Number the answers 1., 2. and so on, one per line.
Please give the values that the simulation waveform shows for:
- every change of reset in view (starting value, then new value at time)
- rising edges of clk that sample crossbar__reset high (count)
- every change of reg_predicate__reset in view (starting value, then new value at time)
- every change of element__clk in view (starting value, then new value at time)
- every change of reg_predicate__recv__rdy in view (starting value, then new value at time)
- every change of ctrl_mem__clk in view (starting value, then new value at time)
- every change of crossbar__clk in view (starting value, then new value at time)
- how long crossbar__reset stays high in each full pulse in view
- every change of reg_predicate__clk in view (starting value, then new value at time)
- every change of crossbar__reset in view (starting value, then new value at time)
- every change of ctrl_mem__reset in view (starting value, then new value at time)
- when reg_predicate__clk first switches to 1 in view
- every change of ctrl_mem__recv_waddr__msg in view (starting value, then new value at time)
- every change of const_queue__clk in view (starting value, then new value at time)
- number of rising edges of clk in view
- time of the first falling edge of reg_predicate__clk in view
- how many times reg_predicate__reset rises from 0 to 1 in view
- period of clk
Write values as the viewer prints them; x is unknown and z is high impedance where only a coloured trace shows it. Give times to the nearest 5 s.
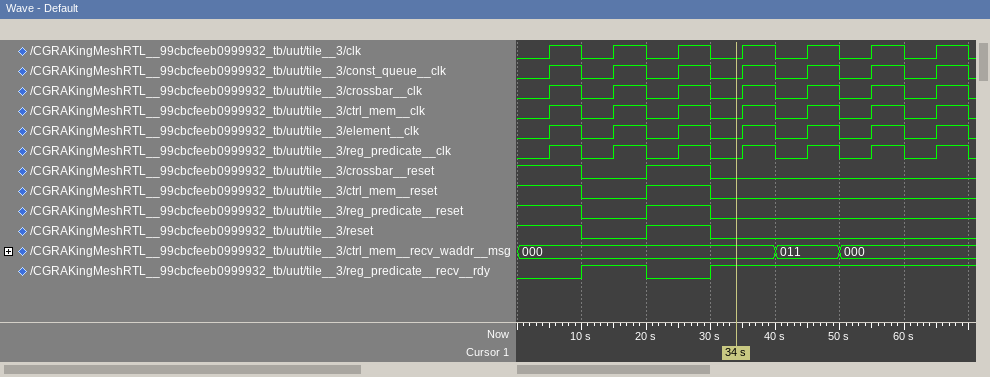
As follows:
1. 1, 0 at 10 s, 1 at 20 s, 0 at 30 s
2. 2
3. 1, 0 at 10 s, 1 at 20 s, 0 at 30 s
4. 0, 1 at 5 s, 0 at 10 s, 1 at 15 s, 0 at 20 s, 1 at 25 s, 0 at 30 s, 1 at 35 s, 0 at 40 s, 1 at 45 s, 0 at 50 s, 1 at 55 s, 0 at 60 s, 1 at 65 s, 0 at 70 s
5. 0, 1 at 10 s, 0 at 20 s, 1 at 30 s
6. 0, 1 at 5 s, 0 at 10 s, 1 at 15 s, 0 at 20 s, 1 at 25 s, 0 at 30 s, 1 at 35 s, 0 at 40 s, 1 at 45 s, 0 at 50 s, 1 at 55 s, 0 at 60 s, 1 at 65 s, 0 at 70 s
7. 0, 1 at 5 s, 0 at 10 s, 1 at 15 s, 0 at 20 s, 1 at 25 s, 0 at 30 s, 1 at 35 s, 0 at 40 s, 1 at 45 s, 0 at 50 s, 1 at 55 s, 0 at 60 s, 1 at 65 s, 0 at 70 s
8. 10 s
9. 0, 1 at 5 s, 0 at 10 s, 1 at 15 s, 0 at 20 s, 1 at 25 s, 0 at 30 s, 1 at 35 s, 0 at 40 s, 1 at 45 s, 0 at 50 s, 1 at 55 s, 0 at 60 s, 1 at 65 s, 0 at 70 s
10. 1, 0 at 10 s, 1 at 20 s, 0 at 30 s
11. 1, 0 at 10 s, 1 at 20 s, 0 at 30 s
12. 5 s
13. 000, 011 at 40 s, 000 at 50 s
14. 0, 1 at 5 s, 0 at 10 s, 1 at 15 s, 0 at 20 s, 1 at 25 s, 0 at 30 s, 1 at 35 s, 0 at 40 s, 1 at 45 s, 0 at 50 s, 1 at 55 s, 0 at 60 s, 1 at 65 s, 0 at 70 s
15. 7
16. 10 s
17. 1
18. 10 s
